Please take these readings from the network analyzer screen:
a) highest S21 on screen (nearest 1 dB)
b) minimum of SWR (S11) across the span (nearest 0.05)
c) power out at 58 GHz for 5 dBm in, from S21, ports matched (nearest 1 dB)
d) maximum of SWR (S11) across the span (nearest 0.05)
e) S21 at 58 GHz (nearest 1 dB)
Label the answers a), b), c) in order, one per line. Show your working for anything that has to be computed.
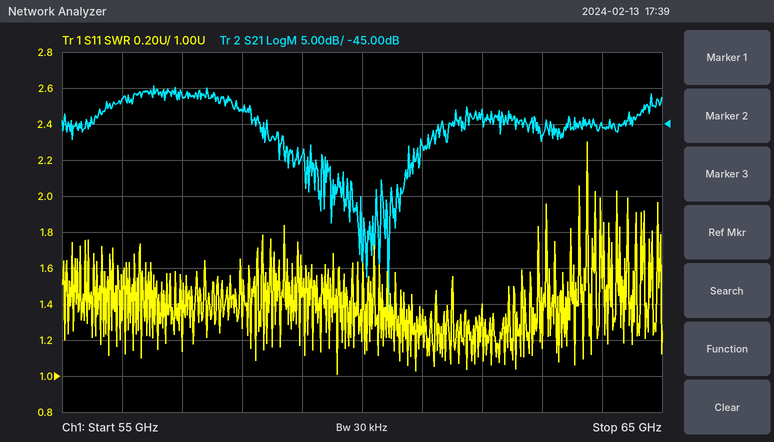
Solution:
a) -40 dB
b) 1.00
c) 5 dBm + (-43 dB) = -38 dBm
d) 2.30
e) -43 dB
